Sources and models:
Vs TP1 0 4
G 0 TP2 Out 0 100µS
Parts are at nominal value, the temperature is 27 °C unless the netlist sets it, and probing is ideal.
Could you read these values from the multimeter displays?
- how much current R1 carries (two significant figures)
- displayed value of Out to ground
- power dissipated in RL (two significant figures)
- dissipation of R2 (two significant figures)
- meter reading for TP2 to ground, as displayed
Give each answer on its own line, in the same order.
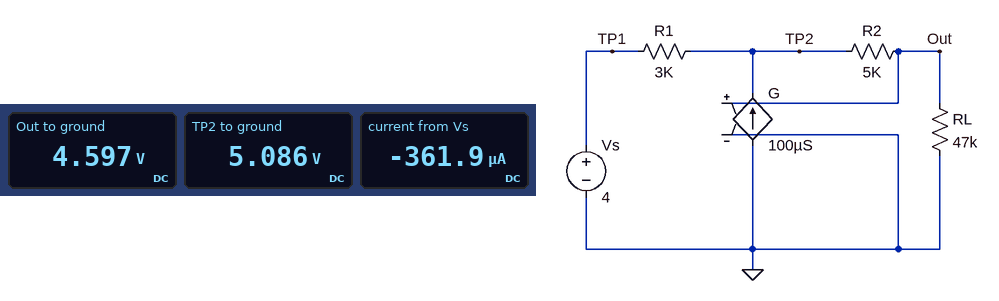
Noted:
360 µA
4.597 V
450 µW
48 µW
5.086 V
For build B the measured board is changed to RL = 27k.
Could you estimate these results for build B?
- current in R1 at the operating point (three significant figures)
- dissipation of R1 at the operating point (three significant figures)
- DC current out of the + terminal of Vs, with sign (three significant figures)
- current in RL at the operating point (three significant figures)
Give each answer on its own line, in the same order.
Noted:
253 µA
192 µW
-253 µA
149 µA
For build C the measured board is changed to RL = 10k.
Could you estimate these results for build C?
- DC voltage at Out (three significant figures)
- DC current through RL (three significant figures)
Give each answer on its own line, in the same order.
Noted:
2.67 V
267 µA
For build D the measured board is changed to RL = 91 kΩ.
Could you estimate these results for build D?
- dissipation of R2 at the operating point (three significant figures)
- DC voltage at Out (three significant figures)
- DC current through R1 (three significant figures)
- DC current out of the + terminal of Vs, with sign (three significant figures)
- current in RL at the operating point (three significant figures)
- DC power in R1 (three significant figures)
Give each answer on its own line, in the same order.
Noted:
15.6 µW
5.08 V
452 µA
-452 µA
55.8 µA
613 µW
